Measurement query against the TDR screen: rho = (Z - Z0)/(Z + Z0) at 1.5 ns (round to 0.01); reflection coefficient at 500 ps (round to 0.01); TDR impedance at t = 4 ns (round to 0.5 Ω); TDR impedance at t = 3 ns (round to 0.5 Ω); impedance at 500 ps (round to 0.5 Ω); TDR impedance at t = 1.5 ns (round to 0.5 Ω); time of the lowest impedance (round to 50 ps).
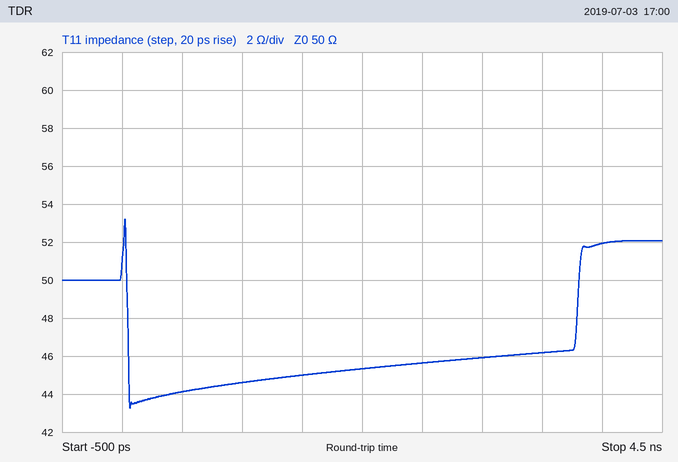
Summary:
-0.05
-0.06
52.0 Ω
46.0 Ω
44.0 Ω
45.0 Ω
50 ps
